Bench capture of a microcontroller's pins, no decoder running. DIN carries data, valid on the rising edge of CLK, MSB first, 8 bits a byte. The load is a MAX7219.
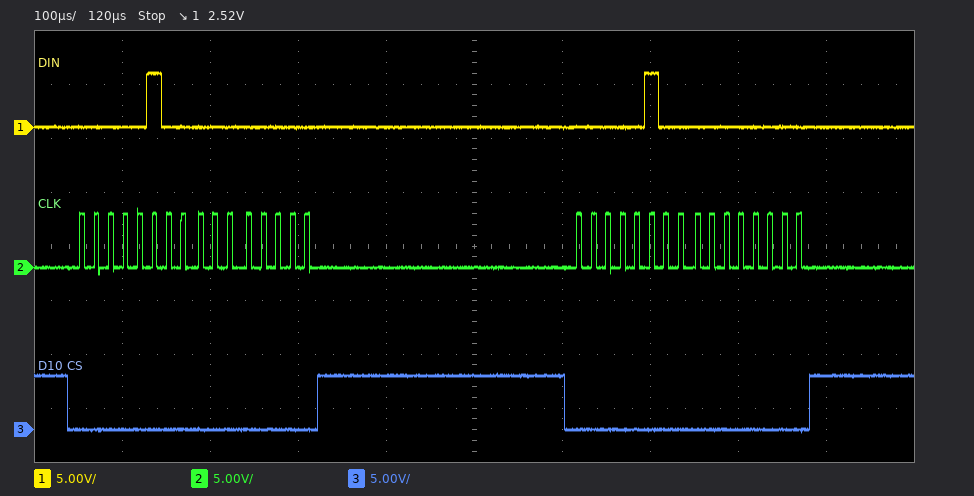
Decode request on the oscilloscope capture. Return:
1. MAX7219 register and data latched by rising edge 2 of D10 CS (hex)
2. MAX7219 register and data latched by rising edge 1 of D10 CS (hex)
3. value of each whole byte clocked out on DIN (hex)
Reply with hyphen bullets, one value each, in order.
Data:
- register 0x4, data 0x00
- register 0x4, data 0x00
- 04 00 04 00
